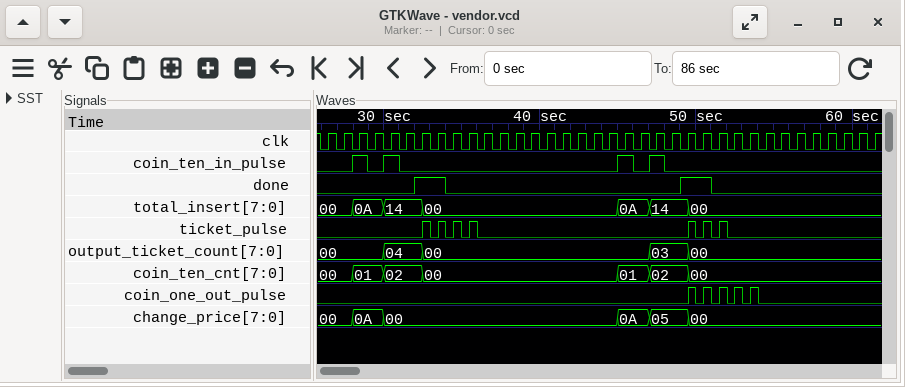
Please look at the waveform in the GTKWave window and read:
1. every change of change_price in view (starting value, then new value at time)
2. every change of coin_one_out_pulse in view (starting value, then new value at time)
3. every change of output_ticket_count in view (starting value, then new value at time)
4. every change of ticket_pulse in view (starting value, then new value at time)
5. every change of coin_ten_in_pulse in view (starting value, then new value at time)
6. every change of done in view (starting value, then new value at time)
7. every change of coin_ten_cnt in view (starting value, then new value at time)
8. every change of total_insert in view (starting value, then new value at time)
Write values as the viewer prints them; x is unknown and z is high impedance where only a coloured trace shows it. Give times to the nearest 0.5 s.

00, 0A at 28 s, 00 at 30 s, 0A at 45 s, 05 at 47 s, 00 at 49.5 s
0, 1 at 49.5 s, 0 at 50 s, 1 at 50.5 s, 0 at 51 s, 1 at 51.5 s, 0 at 52 s, 1 at 52.5 s, 0 at 53 s, 1 at 53.5 s, 0 at 54 s
00, 04 at 30 s, 00 at 32.5 s, 03 at 47 s, 00 at 49.5 s
0, 1 at 32.5 s, 0 at 33 s, 1 at 33.5 s, 0 at 34 s, 1 at 34.5 s, 0 at 35 s, 1 at 35.5 s, 0 at 36 s, 1 at 49.5 s, 0 at 50 s, 1 at 50.5 s, 0 at 51 s, 1 at 51.5 s, 0 at 52 s
0, 1 at 28 s, 0 at 29 s, 1 at 30 s, 0 at 31 s, 1 at 45 s, 0 at 46 s, 1 at 47 s, 0 at 48 s
0, 1 at 32 s, 0 at 34 s, 1 at 49 s, 0 at 51 s
00, 01 at 28 s, 02 at 30 s, 00 at 32.5 s, 01 at 45 s, 02 at 47 s, 00 at 49.5 s
00, 0A at 28 s, 14 at 30 s, 00 at 32.5 s, 0A at 45 s, 14 at 47 s, 00 at 49.5 s
